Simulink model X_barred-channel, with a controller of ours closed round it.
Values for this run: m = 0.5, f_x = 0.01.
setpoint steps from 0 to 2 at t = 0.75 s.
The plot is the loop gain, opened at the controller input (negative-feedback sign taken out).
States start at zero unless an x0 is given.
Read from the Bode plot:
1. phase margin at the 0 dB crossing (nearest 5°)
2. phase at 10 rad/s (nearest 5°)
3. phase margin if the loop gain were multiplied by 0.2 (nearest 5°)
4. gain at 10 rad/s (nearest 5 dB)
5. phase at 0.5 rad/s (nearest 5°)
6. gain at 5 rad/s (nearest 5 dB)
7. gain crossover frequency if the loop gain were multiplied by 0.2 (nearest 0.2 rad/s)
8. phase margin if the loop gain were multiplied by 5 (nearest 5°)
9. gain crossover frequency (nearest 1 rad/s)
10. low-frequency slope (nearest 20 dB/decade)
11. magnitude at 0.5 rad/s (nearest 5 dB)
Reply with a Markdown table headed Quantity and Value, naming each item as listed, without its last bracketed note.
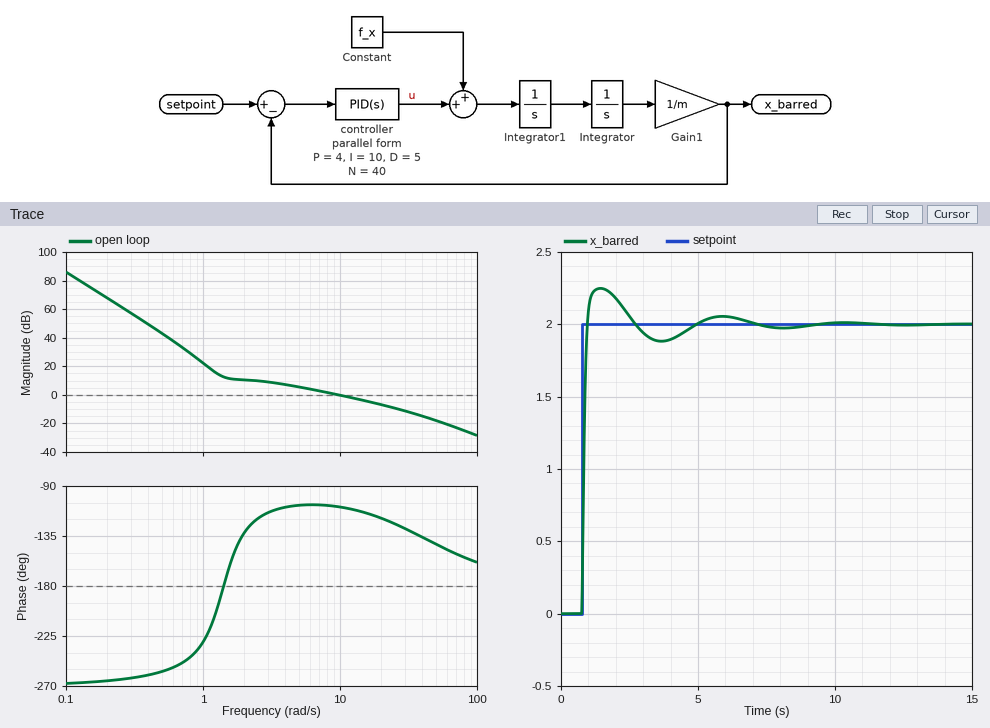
| Quantity | Value |
|---|---|
| phase margin at the 0 dB crossing | 70° |
| phase at 10 rad/s | -110° |
| phase margin if the loop gain were multiplied by 0.2 | -15° |
| gain at 10 rad/s | 0 dB |
| phase at 0.5 rad/s | -255° |
| gain at 5 rad/s | 5 dB |
| gain crossover frequency if the loop gain were multiplied by 0.2 | 1.4 rad/s |
| phase margin if the loop gain were multiplied by 5 | 45° |
| gain crossover frequency | 10 rad/s |
| low-frequency slope | -60 dB/decade |
| magnitude at 0.5 rad/s | 45 dB |
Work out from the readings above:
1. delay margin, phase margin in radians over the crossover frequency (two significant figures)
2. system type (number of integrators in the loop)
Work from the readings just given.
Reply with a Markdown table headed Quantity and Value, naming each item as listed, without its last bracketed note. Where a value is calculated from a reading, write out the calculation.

| Quantity | Value |
|---|---|
| delay margin, phase margin in radians over the crossover frequency | 70 × π / 180 / 10 = 0.12 s |
| system type | 3 |
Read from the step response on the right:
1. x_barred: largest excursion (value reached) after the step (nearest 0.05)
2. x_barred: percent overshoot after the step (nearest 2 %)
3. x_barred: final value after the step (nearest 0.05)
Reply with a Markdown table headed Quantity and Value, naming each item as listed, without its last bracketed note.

| Quantity | Value |
|---|---|
| x_barred: largest excursion (value reached) after the step | 2.25 |
| x_barred: percent overshoot after the step | 12 % |
| x_barred: final value after the step | 2.00 |
